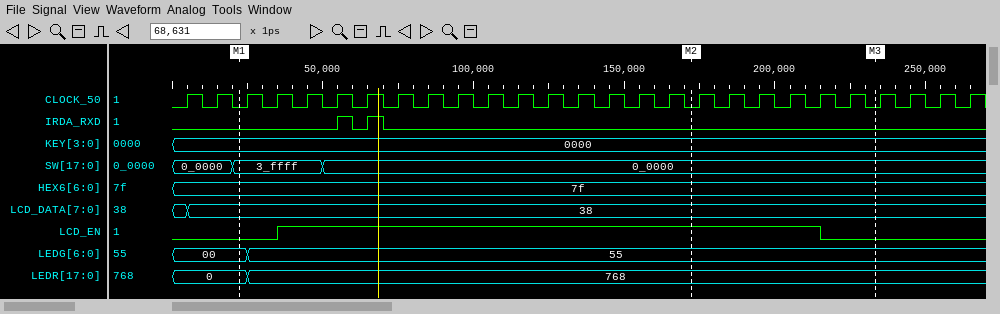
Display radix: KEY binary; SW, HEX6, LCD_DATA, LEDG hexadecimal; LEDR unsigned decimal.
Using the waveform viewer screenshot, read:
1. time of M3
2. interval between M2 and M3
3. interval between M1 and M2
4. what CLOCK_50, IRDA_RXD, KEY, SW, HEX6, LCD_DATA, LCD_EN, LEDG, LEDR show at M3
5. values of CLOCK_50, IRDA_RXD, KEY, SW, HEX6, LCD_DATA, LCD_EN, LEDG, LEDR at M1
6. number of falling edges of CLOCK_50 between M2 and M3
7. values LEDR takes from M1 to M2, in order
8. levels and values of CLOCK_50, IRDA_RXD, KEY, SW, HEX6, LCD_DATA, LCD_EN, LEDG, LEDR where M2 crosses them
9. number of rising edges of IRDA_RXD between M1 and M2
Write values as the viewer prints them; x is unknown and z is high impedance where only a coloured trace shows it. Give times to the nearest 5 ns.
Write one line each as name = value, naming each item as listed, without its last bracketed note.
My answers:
time of M3 = 235 ns
interval between M2 and M3 = 60 ns
interval between M1 and M2 = 150 ns
what CLOCK_50, IRDA_RXD, KEY, SW, HEX6, LCD_DATA, LCD_EN, LEDG, LEDR show at M3 = CLOCK_50=0, IRDA_RXD=0, KEY=0000, SW=0_0000, HEX6=7f, LCD_DATA=38, LCD_EN=0, LEDG=55, LEDR=768
values of CLOCK_50, IRDA_RXD, KEY, SW, HEX6, LCD_DATA, LCD_EN, LEDG, LEDR at M1 = CLOCK_50=0, IRDA_RXD=0, KEY=0000, SW=3_ffff, HEX6=7f, LCD_DATA=38, LCD_EN=0, LEDG=00, LEDR=0
number of falling edges of CLOCK_50 between M2 and M3 = 6
values LEDR takes from M1 to M2, in order = 0, 768
levels and values of CLOCK_50, IRDA_RXD, KEY, SW, HEX6, LCD_DATA, LCD_EN, LEDG, LEDR where M2 crosses them = CLOCK_50=0, IRDA_RXD=0, KEY=0000, SW=0_0000, HEX6=7f, LCD_DATA=38, LCD_EN=1, LEDG=55, LEDR=768
number of rising edges of IRDA_RXD between M1 and M2 = 2
